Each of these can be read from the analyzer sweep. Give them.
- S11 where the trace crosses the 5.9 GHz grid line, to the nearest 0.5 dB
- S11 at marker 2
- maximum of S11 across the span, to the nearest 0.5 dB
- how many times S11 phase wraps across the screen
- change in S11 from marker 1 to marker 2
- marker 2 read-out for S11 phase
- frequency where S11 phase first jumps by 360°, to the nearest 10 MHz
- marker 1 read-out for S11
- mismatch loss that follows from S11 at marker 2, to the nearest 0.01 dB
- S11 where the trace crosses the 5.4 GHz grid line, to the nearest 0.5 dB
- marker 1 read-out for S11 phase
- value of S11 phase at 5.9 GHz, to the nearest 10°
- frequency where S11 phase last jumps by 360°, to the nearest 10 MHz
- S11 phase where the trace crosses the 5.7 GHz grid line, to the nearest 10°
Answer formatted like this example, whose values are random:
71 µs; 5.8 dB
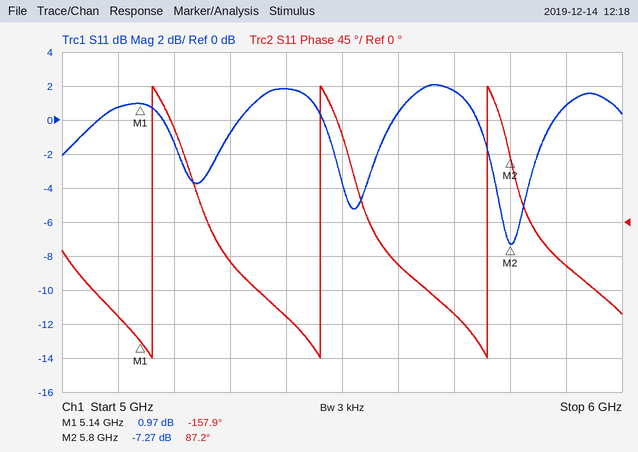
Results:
1.0 dB; -7.27 dB; 2.0 dB; 3; -8.24 dB; 87.2°; 5.16 GHz; 0.97 dB; 0.90 dB; 2.0 dB; -157.9°; -60°; 5.76 GHz; -120°
